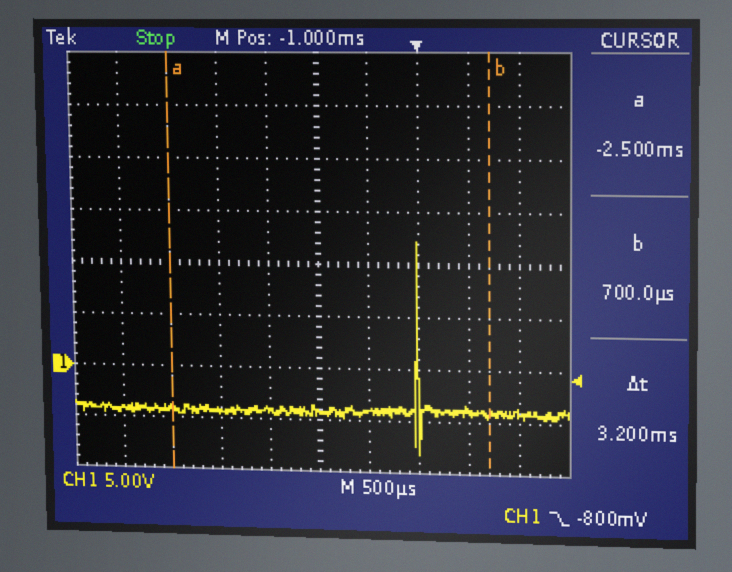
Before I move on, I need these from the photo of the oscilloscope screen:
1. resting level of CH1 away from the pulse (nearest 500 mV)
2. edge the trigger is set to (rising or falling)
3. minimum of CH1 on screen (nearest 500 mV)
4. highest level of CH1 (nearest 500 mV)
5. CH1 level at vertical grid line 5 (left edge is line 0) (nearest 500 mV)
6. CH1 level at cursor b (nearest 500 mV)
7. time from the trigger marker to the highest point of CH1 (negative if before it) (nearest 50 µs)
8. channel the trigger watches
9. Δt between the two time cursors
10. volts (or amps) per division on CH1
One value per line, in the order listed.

-4.0 V
falling
-8.0 V
12.0 V
-4.5 V
-4.0 V
0 µs
CH1
3.2 ms
5 V
